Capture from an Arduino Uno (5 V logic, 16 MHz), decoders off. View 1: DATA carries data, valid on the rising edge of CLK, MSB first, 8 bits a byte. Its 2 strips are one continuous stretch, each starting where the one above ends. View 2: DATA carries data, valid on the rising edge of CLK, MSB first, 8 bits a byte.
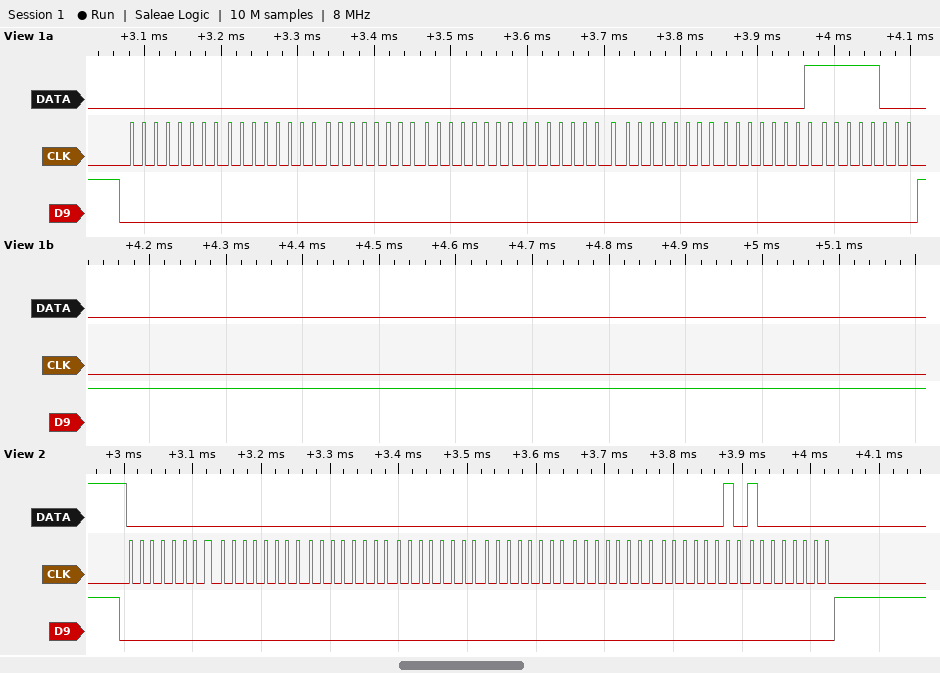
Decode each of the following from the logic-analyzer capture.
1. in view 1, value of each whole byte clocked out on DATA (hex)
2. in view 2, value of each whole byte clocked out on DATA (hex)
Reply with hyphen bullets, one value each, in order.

- 00 00 00 00 00 00 01 F8
- 0x00 0x00 0x00 0x00 0x00 0x00 0x02 0x80
